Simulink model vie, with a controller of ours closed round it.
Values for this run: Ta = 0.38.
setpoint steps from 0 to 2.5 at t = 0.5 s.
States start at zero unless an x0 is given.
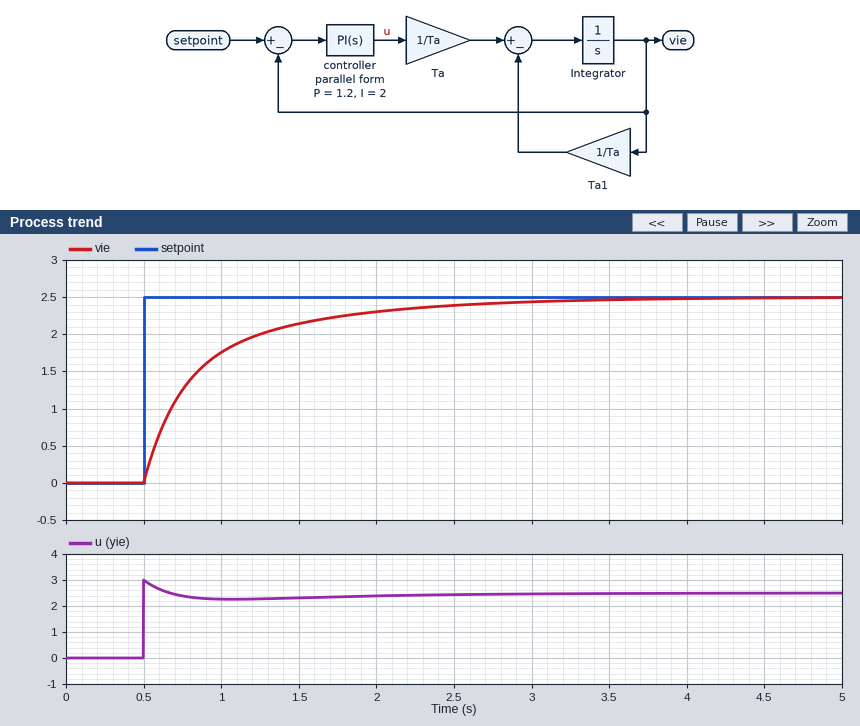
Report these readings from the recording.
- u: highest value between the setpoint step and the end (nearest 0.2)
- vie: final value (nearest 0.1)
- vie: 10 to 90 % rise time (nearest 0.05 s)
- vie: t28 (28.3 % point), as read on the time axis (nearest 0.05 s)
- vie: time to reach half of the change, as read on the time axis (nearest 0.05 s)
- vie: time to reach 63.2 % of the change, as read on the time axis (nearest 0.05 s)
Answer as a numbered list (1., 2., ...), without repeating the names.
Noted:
1. 3.0
2. 2.5
3. 1.25 s
4. 0.60 s
5. 0.75 s
6. 0.90 s
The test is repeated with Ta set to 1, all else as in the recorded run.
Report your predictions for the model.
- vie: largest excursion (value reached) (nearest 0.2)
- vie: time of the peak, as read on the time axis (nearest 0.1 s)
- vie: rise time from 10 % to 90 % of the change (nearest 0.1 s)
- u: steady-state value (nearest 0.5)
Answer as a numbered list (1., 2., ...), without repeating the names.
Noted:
1. 2.6
2. 2.9 s
3. 1.1 s
4. 2.5
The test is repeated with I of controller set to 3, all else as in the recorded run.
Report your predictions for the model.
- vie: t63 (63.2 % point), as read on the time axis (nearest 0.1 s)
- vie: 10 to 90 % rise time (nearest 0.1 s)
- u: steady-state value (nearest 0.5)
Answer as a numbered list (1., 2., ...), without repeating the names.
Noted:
1. 0.8 s
2. 0.7 s
3. 2.5
